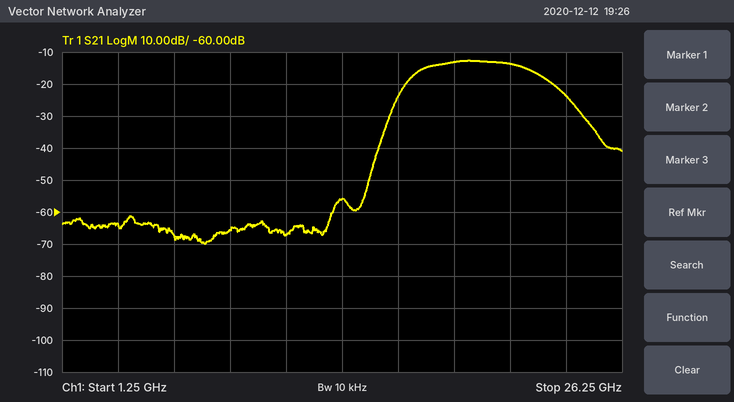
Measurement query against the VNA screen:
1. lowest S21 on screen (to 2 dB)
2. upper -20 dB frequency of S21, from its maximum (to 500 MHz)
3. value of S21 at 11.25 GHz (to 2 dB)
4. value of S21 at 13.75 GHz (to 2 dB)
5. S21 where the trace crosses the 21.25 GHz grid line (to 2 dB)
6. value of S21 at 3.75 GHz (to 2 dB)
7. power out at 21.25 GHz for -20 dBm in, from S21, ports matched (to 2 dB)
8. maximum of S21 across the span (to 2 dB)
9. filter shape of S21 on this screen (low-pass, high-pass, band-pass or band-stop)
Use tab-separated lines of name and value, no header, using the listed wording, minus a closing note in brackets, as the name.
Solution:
lowest S21 on screen	-70 dB
upper -20 dB frequency of S21, from its maximum	25.0 GHz
value of S21 at 11.25 GHz	-68 dB
value of S21 at 13.75 GHz	-56 dB
S21 where the trace crosses the 21.25 GHz grid line	-14 dB
value of S21 at 3.75 GHz	-64 dB
power out at 21.25 GHz for -20 dBm in, from S21, ports matched	-34 dBm
maximum of S21 across the span	-12 dB
filter shape of S21 on this screen	band-pass
